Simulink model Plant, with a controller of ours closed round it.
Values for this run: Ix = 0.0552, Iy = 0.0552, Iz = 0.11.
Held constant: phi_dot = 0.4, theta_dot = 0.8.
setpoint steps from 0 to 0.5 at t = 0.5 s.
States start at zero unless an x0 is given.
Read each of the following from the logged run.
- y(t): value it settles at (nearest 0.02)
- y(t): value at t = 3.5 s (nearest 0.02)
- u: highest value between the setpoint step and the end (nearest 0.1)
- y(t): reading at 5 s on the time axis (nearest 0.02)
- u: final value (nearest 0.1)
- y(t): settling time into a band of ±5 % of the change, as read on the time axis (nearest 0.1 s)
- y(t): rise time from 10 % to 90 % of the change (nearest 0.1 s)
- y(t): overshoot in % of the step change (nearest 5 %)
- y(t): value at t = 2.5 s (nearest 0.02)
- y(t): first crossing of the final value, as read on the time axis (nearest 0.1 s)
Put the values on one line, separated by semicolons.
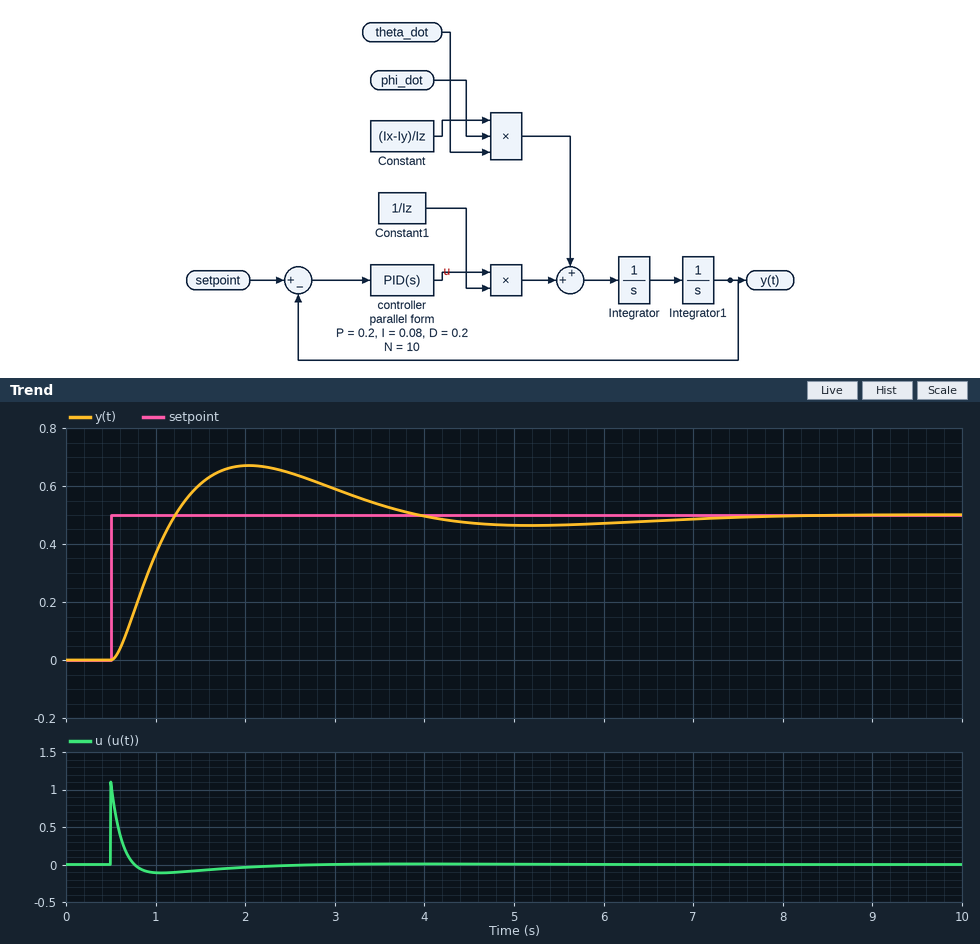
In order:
0.50; 0.54; 1.1; 0.46; 0.0; 6.3 s; 0.5 s; 35 %; 0.64; 1.2 s
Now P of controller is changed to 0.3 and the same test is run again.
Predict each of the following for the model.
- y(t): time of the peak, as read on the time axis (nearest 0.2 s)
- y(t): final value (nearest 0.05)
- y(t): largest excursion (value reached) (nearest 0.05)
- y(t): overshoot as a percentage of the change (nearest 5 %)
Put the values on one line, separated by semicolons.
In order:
1.8 s; 0.50; 0.70; 40 %
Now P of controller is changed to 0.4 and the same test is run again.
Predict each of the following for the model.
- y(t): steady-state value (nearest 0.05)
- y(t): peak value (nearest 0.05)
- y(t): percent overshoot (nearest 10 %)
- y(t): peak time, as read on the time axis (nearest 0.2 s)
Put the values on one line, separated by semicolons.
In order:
0.50; 0.70; 40 %; 1.6 s
